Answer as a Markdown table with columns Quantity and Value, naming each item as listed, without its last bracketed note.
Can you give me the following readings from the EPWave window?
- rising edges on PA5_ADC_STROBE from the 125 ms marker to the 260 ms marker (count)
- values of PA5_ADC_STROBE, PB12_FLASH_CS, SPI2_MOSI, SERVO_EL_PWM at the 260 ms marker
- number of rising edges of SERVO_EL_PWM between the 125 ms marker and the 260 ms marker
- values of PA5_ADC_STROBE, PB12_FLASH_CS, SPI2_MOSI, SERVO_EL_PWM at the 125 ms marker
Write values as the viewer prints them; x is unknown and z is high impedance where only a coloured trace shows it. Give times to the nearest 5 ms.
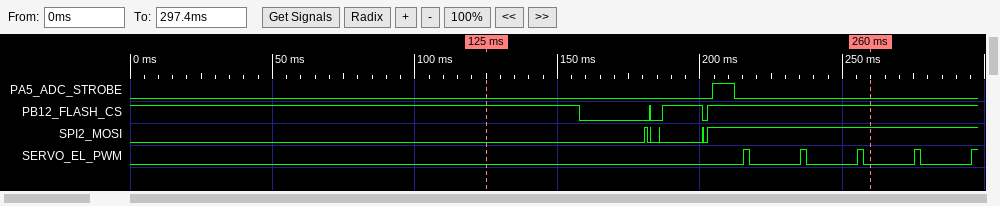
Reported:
| Quantity | Value |
|---|---|
| rising edges on PA5_ADC_STROBE from the 125 ms marker to the 260 ms marker | 1 |
| values of PA5_ADC_STROBE, PB12_FLASH_CS, SPI2_MOSI, SERVO_EL_PWM at the 260 ms marker | PA5_ADC_STROBE=0, PB12_FLASH_CS=1, SPI2_MOSI=1, SERVO_EL_PWM=0 |
| number of rising edges of SERVO_EL_PWM between the 125 ms marker and the 260 ms marker | 3 |
| values of PA5_ADC_STROBE, PB12_FLASH_CS, SPI2_MOSI, SERVO_EL_PWM at the 125 ms marker | PA5_ADC_STROBE=0, PB12_FLASH_CS=1, SPI2_MOSI=0, SERVO_EL_PWM=0 |
